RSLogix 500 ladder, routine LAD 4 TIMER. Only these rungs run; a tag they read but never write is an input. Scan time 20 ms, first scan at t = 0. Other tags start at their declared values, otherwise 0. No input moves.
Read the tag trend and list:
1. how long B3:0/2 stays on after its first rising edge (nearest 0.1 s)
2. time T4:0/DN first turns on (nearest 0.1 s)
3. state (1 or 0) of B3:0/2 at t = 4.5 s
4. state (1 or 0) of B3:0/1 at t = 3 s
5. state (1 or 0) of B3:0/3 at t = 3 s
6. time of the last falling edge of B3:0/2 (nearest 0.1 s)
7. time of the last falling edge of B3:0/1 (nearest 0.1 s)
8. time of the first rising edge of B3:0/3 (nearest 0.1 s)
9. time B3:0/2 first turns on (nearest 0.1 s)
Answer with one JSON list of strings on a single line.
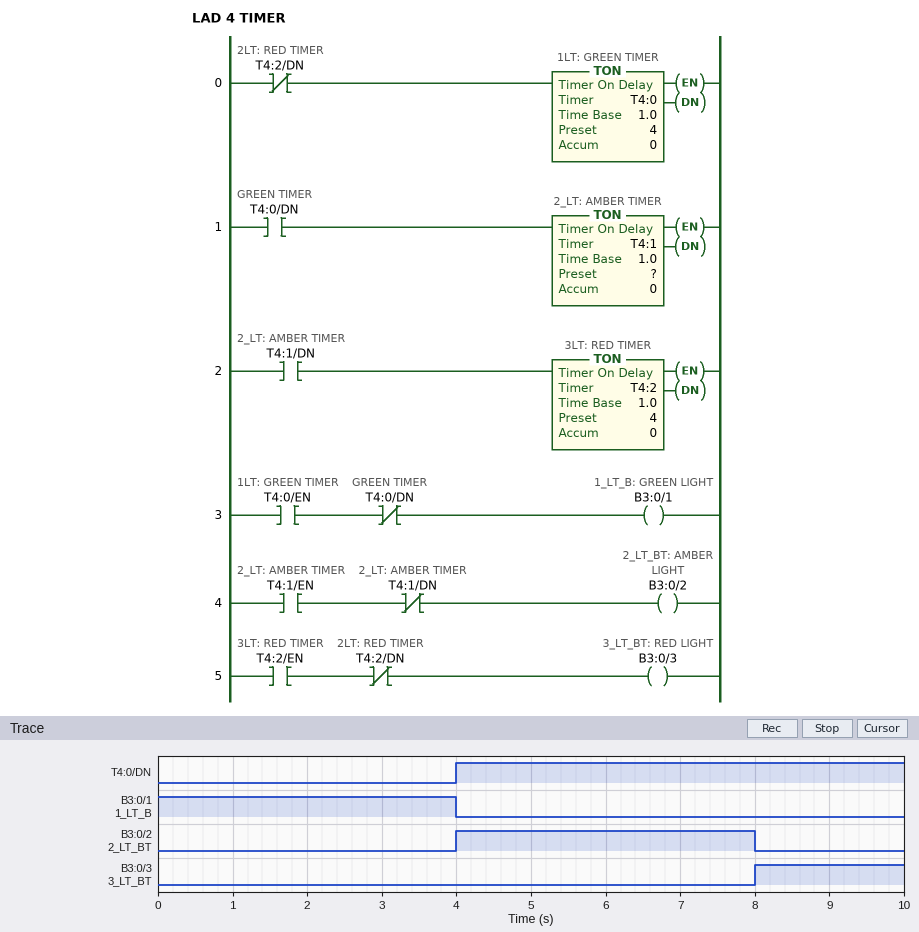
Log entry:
["4.0 s", "4.0 s", "1", "1", "0", "8.0 s", "4.0 s", "8.0 s", "4.0 s"]
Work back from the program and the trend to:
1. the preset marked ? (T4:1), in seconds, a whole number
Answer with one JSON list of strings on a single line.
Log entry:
["4 s"]
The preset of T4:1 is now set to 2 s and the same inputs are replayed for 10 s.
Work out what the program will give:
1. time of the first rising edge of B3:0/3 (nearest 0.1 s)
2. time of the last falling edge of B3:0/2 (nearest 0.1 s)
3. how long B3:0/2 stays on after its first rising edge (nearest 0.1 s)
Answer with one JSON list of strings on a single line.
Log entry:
["6.0 s", "6.0 s", "2.0 s"]
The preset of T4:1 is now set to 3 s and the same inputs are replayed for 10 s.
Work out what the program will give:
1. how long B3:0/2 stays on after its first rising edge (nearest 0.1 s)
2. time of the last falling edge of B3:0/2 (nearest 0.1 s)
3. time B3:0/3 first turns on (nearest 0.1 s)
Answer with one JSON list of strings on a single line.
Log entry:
["3.0 s", "7.0 s", "7.0 s"]
